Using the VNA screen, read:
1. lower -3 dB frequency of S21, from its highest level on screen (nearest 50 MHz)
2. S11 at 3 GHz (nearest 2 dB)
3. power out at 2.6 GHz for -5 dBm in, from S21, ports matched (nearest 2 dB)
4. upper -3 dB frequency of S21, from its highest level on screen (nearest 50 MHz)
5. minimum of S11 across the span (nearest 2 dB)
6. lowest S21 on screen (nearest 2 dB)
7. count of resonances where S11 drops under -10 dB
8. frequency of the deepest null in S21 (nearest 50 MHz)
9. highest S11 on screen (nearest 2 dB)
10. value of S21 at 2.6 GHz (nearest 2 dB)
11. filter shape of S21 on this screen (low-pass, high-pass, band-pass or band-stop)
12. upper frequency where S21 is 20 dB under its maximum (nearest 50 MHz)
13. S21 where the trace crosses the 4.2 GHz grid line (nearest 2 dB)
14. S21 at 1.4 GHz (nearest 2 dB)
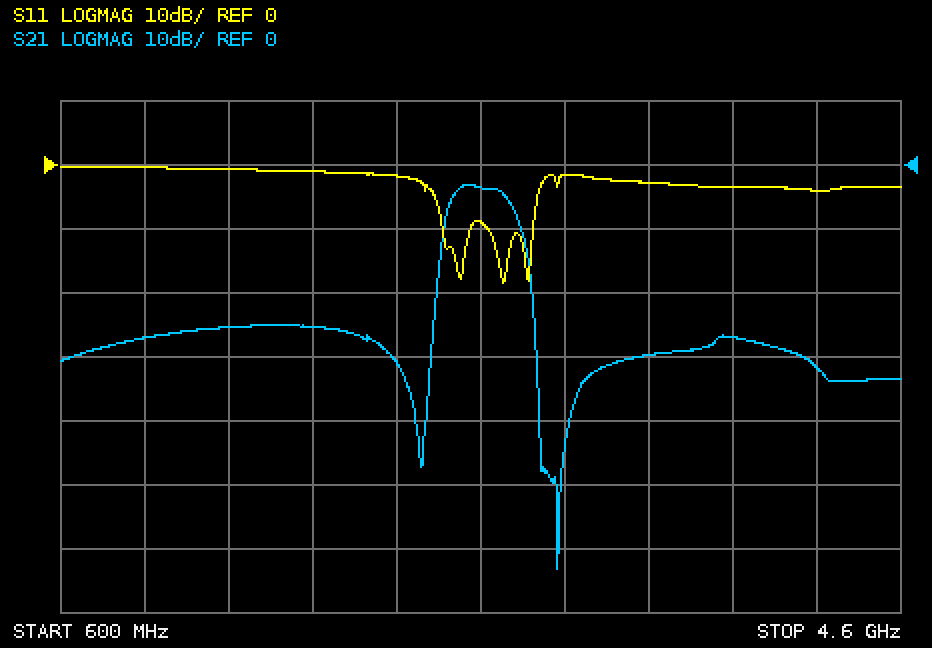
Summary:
2.45 GHz
-2 dB
-8 dBm
2.75 GHz
-18 dB
-64 dB
3
2.95 GHz
0 dB
-4 dB
band-pass
2.85 GHz
-32 dB
-26 dB
